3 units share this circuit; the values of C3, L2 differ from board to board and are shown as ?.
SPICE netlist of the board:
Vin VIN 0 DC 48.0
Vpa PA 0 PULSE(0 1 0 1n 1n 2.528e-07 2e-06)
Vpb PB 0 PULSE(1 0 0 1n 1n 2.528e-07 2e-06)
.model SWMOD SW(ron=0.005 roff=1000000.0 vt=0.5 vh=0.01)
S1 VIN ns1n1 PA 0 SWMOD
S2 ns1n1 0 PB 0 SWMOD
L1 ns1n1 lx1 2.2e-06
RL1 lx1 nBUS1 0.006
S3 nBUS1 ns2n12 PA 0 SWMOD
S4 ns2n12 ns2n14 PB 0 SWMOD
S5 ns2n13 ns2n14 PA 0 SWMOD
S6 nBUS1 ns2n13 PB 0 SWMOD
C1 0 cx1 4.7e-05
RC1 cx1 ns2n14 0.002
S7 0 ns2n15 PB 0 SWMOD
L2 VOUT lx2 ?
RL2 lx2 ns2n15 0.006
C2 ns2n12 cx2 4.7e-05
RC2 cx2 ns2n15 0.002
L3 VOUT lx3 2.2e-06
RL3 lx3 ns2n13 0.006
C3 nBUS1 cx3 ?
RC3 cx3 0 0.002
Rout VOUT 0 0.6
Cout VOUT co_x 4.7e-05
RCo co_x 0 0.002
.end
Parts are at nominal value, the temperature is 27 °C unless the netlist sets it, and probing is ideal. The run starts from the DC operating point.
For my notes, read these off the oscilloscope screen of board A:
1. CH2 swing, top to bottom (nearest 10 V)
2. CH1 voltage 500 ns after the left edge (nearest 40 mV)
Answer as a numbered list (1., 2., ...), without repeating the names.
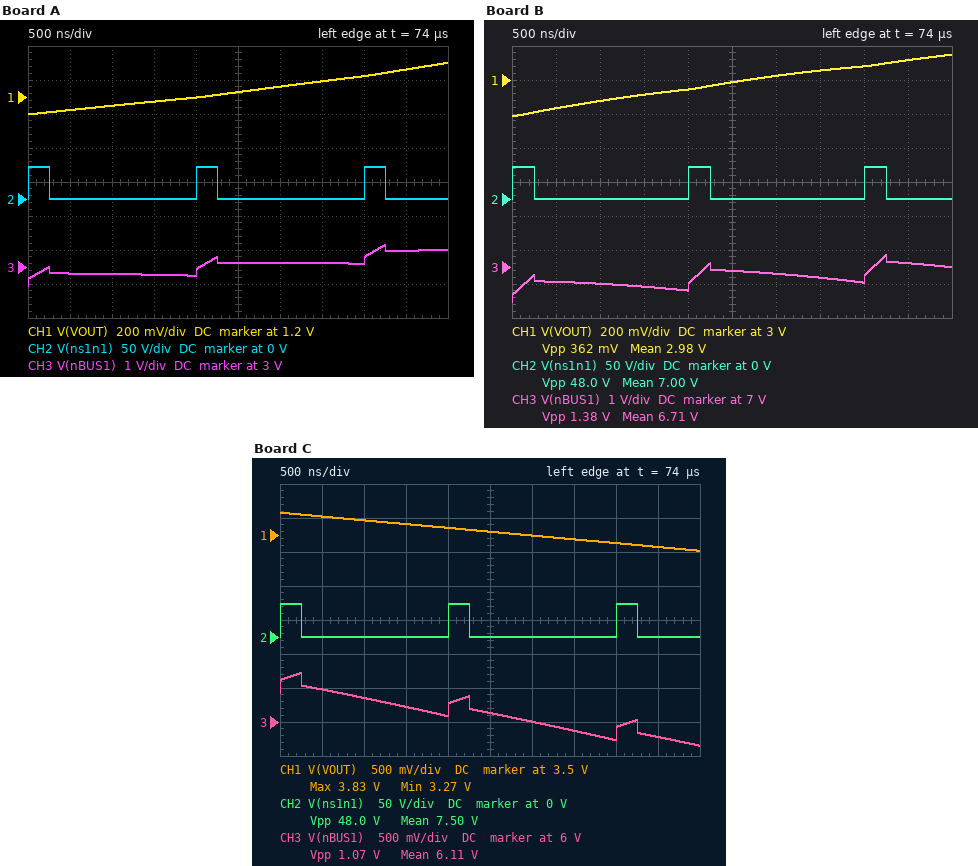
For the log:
1. 50 V
2. 1.12 V
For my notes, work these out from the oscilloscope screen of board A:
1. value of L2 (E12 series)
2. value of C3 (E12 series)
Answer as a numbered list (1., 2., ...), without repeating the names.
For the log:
1. 1.2 µH
2. 68 µF
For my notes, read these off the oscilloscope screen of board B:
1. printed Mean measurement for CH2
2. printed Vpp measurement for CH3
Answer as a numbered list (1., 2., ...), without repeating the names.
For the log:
1. 7.00 V
2. 1.38 V
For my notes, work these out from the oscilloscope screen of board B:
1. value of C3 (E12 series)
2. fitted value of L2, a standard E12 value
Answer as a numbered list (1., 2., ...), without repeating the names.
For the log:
1. 39 µF
2. 1 µH
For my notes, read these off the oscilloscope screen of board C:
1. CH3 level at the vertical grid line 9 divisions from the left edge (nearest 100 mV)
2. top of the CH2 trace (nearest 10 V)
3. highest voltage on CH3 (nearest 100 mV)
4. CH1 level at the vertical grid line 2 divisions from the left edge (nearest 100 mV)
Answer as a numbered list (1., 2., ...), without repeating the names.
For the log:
1. 5.8 V
2. 50 V
3. 6.7 V
4. 3.7 V
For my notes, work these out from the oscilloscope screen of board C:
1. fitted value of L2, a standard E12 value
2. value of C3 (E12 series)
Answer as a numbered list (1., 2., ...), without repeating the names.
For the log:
1. 3.3 µH
2. 150 µF
